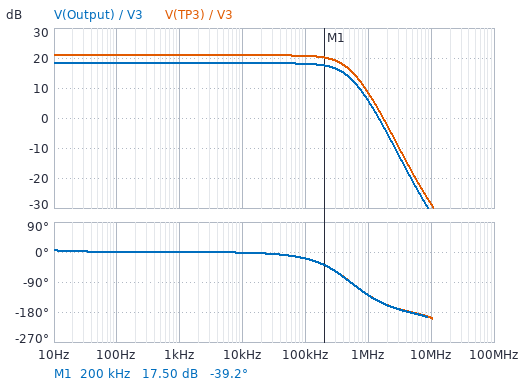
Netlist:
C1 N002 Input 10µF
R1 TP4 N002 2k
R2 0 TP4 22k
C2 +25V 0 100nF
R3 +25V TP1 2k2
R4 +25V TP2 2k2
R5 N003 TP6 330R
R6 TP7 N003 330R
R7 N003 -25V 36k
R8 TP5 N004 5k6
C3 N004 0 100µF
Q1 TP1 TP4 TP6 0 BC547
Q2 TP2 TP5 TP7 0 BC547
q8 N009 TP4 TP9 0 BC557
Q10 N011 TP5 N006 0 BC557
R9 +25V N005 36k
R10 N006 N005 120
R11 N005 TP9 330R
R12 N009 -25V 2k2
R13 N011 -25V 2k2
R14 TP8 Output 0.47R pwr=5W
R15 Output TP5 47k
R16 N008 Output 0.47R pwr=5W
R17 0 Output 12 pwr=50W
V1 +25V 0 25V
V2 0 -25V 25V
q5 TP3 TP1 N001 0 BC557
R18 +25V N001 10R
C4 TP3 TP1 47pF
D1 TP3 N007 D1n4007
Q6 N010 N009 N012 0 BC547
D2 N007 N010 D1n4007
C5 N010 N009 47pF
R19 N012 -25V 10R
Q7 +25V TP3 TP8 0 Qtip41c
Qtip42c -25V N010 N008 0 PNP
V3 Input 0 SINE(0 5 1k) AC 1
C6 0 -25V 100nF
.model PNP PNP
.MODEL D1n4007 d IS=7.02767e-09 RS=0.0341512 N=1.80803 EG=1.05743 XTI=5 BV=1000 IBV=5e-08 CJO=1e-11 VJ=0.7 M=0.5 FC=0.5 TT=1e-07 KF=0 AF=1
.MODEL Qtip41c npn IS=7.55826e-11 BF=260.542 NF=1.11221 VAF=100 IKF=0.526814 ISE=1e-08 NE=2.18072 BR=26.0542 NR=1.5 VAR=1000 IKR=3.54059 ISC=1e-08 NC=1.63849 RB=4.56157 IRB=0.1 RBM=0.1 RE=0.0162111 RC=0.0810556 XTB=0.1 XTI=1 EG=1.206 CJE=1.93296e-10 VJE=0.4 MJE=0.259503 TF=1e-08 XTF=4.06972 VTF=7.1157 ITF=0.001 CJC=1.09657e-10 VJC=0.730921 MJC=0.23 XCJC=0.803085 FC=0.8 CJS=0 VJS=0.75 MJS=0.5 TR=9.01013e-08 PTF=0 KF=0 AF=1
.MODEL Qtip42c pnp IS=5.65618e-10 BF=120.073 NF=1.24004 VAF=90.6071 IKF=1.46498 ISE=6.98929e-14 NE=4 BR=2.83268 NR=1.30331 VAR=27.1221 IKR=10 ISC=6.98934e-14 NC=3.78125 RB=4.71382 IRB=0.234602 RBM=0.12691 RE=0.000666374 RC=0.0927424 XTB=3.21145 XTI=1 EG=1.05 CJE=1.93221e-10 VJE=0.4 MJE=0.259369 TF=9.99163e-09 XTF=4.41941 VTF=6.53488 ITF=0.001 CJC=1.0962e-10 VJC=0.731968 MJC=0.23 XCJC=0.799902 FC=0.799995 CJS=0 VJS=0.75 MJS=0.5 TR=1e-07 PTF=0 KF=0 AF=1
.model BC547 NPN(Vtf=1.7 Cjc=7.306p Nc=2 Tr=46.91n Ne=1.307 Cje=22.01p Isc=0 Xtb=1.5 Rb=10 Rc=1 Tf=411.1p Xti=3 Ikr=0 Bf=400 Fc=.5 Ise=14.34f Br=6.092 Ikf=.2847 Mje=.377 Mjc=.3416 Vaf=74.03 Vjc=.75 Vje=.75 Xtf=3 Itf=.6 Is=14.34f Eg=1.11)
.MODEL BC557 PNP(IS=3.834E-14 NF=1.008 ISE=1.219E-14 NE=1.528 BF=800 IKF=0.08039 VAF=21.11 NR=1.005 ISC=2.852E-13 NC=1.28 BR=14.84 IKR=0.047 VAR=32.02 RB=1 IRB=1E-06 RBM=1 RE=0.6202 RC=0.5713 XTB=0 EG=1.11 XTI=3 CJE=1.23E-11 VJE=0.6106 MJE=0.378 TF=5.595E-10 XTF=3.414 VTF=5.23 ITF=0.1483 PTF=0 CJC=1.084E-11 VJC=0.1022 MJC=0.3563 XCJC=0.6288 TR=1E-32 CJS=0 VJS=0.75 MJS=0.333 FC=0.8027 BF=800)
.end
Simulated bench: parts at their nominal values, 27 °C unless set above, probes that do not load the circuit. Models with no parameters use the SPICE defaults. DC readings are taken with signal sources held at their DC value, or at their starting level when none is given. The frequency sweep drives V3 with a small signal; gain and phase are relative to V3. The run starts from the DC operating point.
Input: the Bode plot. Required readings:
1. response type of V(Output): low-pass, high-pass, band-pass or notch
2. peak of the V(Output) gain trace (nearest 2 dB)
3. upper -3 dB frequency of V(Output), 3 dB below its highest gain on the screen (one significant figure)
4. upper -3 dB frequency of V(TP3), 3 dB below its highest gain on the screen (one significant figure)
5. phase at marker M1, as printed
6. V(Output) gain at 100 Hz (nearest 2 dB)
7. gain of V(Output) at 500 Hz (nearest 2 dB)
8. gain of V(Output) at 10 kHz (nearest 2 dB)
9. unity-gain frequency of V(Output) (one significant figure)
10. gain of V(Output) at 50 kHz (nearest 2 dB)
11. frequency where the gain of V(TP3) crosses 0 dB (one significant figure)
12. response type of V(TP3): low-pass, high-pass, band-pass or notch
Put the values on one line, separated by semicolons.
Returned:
low-pass; 18 dB; 400 kHz; 400 kHz; -39.2 deg; 18 dB; 18 dB; 18 dB; 1 MHz; 18 dB; 2 MHz; low-pass
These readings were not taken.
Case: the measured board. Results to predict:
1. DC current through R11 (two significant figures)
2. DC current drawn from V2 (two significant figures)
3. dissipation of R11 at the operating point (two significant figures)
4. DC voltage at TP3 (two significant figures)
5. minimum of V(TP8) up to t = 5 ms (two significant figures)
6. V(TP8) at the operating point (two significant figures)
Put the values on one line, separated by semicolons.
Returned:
300 µA; 2.2 mA; 29 µW; 620 mV; -23 V; 98 mV
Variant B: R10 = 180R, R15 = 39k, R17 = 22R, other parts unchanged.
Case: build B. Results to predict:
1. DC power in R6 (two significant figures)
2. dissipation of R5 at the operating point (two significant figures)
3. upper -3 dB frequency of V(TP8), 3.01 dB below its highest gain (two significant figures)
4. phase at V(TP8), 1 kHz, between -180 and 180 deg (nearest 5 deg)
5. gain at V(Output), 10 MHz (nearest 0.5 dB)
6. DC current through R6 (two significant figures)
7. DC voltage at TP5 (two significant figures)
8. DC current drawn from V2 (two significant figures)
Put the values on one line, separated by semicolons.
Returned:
47 µW; 29 µW; 450 kHz; 0 deg; -27.0 dB; 380 µA; 6.9 mV; 3.2 mA
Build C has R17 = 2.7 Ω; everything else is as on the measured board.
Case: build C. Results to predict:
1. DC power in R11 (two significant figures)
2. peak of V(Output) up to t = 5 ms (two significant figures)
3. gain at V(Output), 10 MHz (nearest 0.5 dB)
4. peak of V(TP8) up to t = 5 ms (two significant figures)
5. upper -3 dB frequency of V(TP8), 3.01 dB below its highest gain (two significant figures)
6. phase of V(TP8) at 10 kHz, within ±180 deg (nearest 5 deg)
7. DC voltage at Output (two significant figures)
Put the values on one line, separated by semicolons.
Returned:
28 µW; 8.8 V; -42.0 dB; 10 V; 260 kHz; -5 deg; 92 mV
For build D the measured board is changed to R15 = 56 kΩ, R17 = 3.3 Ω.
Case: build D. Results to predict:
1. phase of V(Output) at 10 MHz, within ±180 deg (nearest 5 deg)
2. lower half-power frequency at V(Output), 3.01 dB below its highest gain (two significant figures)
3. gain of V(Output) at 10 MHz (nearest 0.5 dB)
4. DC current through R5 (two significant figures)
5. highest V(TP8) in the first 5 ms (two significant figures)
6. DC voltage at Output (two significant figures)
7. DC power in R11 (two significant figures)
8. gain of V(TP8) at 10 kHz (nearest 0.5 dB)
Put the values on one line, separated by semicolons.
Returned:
150 deg; 750 mHz; -40.5 dB; 280 µA; 12 V; 110 mV; 28 µW; 20.0 dB
